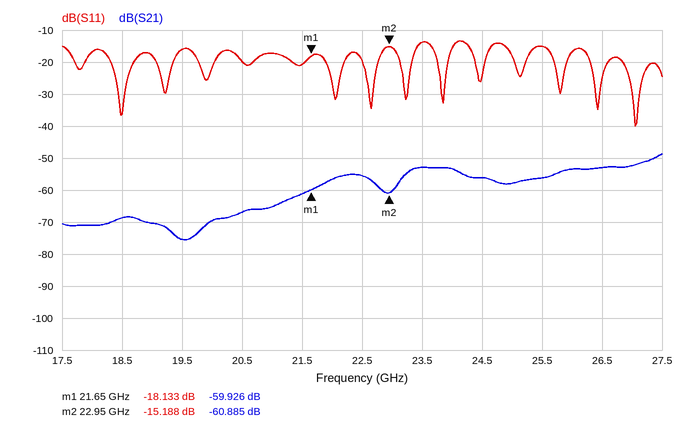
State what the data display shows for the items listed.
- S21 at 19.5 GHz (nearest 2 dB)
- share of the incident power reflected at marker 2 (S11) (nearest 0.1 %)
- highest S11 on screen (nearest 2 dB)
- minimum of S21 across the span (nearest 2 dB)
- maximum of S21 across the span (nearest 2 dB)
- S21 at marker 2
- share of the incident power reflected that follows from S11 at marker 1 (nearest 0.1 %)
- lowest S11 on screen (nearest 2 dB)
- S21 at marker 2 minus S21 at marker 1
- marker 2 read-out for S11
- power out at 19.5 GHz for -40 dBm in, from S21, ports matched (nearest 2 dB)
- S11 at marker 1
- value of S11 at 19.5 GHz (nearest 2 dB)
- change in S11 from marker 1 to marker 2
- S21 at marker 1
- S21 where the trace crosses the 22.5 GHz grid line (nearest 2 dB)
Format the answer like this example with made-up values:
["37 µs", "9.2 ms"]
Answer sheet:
["-76 dB", "3.0 %", "-14 dB", "-76 dB", "-48 dB", "-60.885 dB", "1.5 %", "-40 dB", "-0.959 dB", "-15.188 dB", "-116 dBm", "-18.133 dB", "-16 dB", "2.945 dB", "-59.926 dB", "-56 dB"]
